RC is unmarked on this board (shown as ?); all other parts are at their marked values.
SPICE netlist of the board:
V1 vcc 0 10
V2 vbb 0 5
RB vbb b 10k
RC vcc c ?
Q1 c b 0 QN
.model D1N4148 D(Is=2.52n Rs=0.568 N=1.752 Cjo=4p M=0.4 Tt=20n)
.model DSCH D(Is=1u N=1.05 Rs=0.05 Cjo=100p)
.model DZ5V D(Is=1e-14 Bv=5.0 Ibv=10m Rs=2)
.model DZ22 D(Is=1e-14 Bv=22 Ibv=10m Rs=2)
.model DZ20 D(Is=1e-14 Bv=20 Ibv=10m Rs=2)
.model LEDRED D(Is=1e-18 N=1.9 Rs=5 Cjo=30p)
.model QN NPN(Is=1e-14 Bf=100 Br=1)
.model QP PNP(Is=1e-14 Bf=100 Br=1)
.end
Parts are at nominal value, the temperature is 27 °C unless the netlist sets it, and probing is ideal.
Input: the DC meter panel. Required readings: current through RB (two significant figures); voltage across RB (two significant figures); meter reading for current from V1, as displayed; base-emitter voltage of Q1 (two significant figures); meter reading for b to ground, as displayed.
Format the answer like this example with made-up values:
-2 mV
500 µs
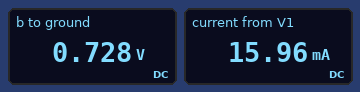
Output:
430 µA
4.3 V
15.96 mA
730 mV
0.728 V
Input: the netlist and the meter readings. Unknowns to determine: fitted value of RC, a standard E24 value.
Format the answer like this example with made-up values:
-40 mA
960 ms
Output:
620 Ω
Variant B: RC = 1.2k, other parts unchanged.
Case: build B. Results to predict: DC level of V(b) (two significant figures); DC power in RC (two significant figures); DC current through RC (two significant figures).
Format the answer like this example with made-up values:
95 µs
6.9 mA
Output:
710 mV
82 mW
8.3 mA
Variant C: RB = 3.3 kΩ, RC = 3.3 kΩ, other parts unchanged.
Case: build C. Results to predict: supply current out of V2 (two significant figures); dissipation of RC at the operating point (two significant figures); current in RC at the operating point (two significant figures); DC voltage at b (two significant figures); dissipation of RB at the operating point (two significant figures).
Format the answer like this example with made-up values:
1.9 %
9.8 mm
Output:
1.3 mA
30 mW
3.0 mA
700 mV
5.6 mW
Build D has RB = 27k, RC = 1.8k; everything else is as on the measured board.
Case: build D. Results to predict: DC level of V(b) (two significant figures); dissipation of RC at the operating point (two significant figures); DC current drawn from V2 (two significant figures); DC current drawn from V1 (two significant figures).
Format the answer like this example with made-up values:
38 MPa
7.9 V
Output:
700 mV
54 mW
160 µA
5.5 mA
